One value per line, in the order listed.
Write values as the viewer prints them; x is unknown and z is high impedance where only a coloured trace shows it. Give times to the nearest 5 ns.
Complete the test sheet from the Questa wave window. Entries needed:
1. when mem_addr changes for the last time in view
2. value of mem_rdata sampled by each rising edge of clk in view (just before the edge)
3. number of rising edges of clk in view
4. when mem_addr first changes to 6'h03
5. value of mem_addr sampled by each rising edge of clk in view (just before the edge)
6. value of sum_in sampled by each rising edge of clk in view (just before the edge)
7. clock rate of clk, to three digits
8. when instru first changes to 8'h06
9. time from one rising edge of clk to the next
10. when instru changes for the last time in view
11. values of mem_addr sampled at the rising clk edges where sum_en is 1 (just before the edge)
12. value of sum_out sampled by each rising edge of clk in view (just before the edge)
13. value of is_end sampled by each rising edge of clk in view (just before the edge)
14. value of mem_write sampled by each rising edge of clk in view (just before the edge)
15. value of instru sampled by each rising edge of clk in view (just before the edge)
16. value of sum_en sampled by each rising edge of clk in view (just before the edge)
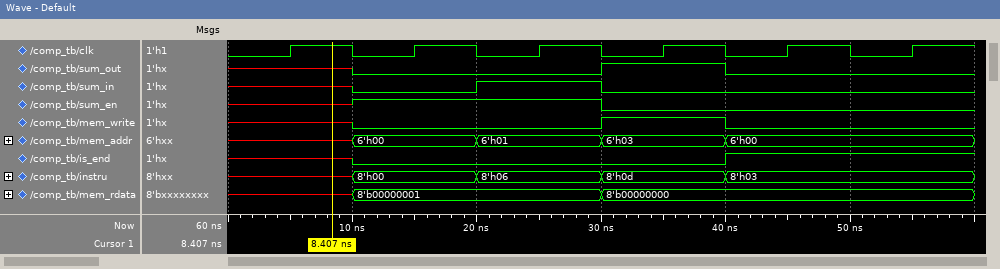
40 ns
x, 8'b00000001, 8'b00000001, 8'b00000000, 8'b00000000, 8'b00000000
6
30 ns
x, 6'h00, 6'h01, 6'h03, 6'h00, 6'h00
x 0 1 0 0 0
100 MHz
20 ns
10 ns
40 ns
6'h00, 6'h01
x 0 0 1 0 0
x 0 0 0 1 1
x 0 0 1 0 0
x, 8'h00, 8'h06, 8'h0d, 8'h03, 8'h03
x 1 1 0 0 0
